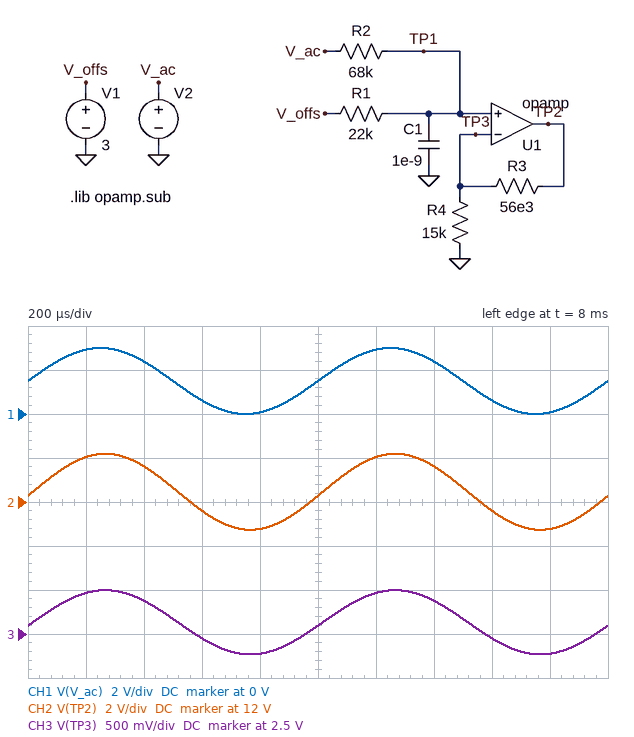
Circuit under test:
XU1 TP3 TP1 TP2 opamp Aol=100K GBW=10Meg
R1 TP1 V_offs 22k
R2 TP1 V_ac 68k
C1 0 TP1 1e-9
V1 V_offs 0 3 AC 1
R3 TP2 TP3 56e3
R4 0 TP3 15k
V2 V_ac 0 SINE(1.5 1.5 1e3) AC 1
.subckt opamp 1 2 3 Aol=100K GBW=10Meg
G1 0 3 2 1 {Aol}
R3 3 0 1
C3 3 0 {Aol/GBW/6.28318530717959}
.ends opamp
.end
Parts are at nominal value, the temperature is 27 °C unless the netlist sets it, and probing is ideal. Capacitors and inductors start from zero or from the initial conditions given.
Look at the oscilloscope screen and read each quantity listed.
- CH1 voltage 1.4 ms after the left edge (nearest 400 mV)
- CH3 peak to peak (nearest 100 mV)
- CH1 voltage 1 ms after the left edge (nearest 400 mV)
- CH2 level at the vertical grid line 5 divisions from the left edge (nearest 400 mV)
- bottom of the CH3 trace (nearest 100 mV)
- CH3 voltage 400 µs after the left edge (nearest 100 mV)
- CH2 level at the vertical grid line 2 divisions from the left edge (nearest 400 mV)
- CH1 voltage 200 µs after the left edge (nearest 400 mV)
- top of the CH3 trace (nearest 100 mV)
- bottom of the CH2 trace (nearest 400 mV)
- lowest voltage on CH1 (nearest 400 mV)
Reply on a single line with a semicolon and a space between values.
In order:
2.4 V; 700 mV; 1.6 V; 12.4 V; 2.3 V; 2.9 V; 13.6 V; 2.8 V; 3.0 V; 10.8 V; 0 V
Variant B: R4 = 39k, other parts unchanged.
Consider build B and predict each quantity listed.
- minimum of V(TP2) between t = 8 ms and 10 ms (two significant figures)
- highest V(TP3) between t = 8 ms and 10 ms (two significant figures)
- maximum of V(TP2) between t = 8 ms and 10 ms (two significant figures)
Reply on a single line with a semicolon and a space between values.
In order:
5.5 V; 3.0 V; 7.3 V
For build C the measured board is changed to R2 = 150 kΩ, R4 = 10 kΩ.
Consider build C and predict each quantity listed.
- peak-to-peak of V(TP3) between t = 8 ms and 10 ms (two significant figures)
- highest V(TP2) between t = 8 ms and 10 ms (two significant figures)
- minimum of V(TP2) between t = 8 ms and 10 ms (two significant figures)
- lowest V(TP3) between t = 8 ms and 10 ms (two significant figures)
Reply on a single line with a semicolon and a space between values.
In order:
380 mV; 20 V; 17 V; 2.6 V
